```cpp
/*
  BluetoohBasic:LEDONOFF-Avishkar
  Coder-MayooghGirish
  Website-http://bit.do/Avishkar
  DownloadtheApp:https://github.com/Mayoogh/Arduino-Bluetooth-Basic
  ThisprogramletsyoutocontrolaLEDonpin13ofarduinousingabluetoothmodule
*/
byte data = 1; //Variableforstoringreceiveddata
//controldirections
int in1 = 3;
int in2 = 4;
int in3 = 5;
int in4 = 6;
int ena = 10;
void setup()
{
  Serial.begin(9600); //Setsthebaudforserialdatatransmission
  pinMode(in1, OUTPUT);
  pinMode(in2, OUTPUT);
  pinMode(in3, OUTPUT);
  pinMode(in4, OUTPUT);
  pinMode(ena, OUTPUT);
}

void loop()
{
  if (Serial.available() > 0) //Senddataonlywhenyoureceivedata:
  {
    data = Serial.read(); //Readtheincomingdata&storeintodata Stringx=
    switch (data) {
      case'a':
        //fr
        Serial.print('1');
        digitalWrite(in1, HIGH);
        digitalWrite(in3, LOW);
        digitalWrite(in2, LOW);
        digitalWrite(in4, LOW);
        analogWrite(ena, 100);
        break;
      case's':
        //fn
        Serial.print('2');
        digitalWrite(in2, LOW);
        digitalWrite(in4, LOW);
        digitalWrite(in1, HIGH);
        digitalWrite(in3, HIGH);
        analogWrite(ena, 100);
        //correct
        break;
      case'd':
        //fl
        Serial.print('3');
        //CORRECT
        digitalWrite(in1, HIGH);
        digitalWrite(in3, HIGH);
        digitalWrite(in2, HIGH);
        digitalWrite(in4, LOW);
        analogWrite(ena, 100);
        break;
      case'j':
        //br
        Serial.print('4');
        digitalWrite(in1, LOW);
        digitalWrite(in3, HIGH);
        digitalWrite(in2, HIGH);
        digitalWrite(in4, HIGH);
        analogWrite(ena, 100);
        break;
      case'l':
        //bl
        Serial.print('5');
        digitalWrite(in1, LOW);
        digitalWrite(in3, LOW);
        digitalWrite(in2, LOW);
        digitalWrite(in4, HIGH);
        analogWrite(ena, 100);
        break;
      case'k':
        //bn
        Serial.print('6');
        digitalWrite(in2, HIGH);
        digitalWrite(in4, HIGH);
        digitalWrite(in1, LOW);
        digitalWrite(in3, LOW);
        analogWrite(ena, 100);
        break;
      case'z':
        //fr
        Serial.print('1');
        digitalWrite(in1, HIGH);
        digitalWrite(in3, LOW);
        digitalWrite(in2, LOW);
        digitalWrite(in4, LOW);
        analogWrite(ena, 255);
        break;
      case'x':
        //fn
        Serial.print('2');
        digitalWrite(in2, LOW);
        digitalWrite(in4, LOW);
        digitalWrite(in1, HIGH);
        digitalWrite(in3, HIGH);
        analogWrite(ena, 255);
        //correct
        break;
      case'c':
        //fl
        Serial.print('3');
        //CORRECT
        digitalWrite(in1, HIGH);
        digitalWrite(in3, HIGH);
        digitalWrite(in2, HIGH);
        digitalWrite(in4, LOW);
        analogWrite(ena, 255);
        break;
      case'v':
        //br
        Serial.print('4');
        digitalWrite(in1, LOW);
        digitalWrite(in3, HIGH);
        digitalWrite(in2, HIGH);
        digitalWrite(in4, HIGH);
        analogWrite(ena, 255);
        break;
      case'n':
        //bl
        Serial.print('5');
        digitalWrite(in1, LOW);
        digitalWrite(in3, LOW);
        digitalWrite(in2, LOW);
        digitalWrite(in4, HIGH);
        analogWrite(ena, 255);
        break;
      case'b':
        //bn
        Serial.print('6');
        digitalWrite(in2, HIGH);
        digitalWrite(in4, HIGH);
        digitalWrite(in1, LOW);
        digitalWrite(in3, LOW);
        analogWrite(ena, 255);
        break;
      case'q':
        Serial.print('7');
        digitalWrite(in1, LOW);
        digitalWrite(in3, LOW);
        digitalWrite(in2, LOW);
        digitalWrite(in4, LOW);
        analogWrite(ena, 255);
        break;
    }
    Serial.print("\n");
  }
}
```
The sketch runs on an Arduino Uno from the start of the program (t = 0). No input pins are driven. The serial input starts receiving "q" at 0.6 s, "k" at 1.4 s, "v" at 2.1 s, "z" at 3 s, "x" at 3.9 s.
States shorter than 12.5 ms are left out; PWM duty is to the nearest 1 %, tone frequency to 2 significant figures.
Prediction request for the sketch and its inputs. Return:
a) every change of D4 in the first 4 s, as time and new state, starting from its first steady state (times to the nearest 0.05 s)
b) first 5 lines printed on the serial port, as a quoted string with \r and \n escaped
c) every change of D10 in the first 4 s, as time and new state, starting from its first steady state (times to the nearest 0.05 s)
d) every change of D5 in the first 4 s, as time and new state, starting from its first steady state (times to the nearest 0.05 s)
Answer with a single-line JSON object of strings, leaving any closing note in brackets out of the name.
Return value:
{"every change of D4 in the first 4 s, as time and new state, starting from its first steady state": "0 s low; 1.4 s high; 3 s low", "first 5 lines printed on the serial port, as a quoted string with \\r and \\n escaped": "\"7\\n6\\n4\\n1\\n2\\n\"", "every change of D10 in the first 4 s, as time and new state, starting from its first steady state": "0 s low; 0.6 s high; 1.4 s PWM 39 %; 2.1 s high", "every change of D5 in the first 4 s, as time and new state, starting from its first steady state": "0 s low; 2.1 s high; 3 s low; 3.9 s high"}
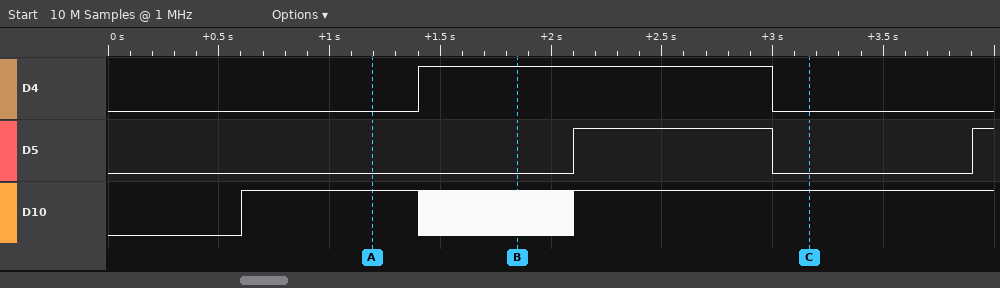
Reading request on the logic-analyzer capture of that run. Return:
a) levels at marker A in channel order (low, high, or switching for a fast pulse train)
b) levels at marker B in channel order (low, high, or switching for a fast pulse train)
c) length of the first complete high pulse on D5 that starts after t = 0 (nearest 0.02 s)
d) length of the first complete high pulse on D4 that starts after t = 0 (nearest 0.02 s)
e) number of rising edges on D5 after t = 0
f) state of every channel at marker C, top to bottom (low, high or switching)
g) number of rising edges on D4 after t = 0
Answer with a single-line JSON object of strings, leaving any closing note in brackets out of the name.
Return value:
{"levels at marker A in channel order": "D4 low, D5 low, D10 high", "levels at marker B in channel order": "D4 high, D5 low, D10 switching", "length of the first complete high pulse on D5 that starts after t = 0": "0.90 s", "length of the first complete high pulse on D4 that starts after t = 0": "1.60 s", "number of rising edges on D5 after t = 0": "2", "state of every channel at marker C, top to bottom": "D4 low, D5 low, D10 high", "number of rising edges on D4 after t = 0": "1"}
